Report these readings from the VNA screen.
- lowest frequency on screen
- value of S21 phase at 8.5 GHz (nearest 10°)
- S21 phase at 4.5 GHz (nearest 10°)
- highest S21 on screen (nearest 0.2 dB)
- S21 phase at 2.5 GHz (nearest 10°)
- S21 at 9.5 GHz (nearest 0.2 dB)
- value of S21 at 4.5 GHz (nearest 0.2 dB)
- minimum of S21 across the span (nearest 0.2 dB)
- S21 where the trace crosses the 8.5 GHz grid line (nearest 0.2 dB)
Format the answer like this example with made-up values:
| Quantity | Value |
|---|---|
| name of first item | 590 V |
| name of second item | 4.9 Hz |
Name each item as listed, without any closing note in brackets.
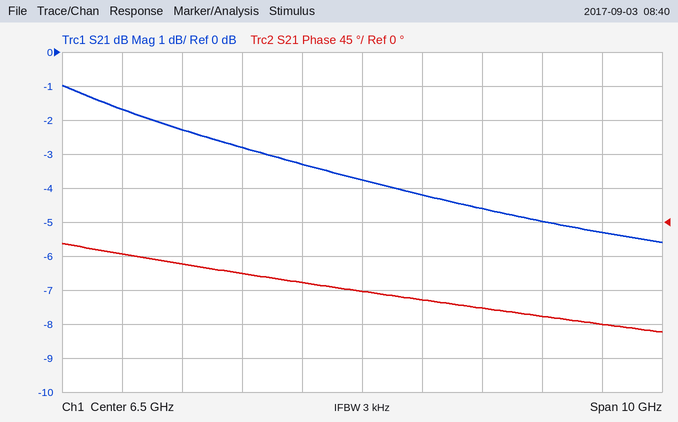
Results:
| Quantity | Value |
|---|---|
| lowest frequency on screen | 1.5 GHz |
| value of S21 phase at 8.5 GHz | -110° |
| S21 phase at 4.5 GHz | -70° |
| highest S21 on screen | -1.0 dB |
| S21 phase at 2.5 GHz | -40° |
| S21 at 9.5 GHz | -5.0 dB |
| value of S21 at 4.5 GHz | -2.8 dB |
| minimum of S21 across the span | -5.6 dB |
| S21 where the trace crosses the 8.5 GHz grid line | -4.6 dB |
